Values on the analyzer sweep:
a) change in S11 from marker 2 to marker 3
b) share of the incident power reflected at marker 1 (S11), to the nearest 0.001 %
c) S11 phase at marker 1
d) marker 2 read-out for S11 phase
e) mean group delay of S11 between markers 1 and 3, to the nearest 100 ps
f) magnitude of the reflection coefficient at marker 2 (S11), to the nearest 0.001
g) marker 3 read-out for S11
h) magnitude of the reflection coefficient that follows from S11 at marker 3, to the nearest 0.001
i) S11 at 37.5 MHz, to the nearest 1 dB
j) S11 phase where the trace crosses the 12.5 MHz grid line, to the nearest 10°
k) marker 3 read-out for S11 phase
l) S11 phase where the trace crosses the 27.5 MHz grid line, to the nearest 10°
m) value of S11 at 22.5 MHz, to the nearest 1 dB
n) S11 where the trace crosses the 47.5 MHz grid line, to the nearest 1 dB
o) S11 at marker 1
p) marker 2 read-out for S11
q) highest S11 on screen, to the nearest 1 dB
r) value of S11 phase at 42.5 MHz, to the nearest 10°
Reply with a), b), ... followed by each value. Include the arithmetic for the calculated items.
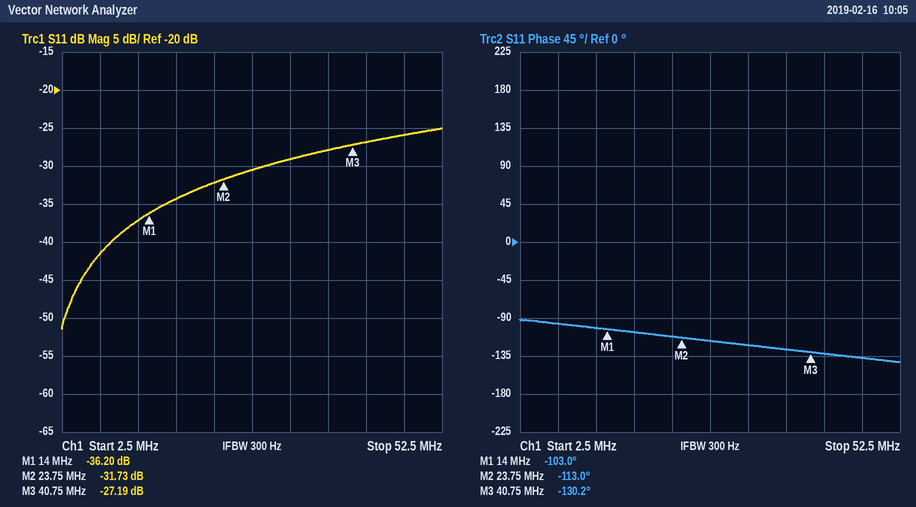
a) -27.19 − (-31.73) = 4.54 dB
b) 10^(-36.2/10) ≈ 0.024 %
c) -103.0°
d) -113.0°
e) −(-130.2° − (-103°))/(360° × 26.75 MHz) ≈ 2.8 ns
f) 10^(-31.73/20) ≈ 0.026
g) -27.19 dB
h) 10^(-27.19/20) ≈ 0.044
i) -28 dB
j) -100°
k) -130.2°
l) -120°
m) -32 dB
n) -26 dB
o) -36.20 dB
p) -31.73 dB
q) -25 dB
r) -130°
